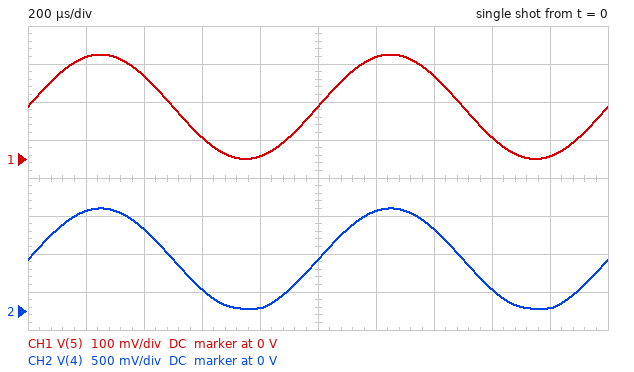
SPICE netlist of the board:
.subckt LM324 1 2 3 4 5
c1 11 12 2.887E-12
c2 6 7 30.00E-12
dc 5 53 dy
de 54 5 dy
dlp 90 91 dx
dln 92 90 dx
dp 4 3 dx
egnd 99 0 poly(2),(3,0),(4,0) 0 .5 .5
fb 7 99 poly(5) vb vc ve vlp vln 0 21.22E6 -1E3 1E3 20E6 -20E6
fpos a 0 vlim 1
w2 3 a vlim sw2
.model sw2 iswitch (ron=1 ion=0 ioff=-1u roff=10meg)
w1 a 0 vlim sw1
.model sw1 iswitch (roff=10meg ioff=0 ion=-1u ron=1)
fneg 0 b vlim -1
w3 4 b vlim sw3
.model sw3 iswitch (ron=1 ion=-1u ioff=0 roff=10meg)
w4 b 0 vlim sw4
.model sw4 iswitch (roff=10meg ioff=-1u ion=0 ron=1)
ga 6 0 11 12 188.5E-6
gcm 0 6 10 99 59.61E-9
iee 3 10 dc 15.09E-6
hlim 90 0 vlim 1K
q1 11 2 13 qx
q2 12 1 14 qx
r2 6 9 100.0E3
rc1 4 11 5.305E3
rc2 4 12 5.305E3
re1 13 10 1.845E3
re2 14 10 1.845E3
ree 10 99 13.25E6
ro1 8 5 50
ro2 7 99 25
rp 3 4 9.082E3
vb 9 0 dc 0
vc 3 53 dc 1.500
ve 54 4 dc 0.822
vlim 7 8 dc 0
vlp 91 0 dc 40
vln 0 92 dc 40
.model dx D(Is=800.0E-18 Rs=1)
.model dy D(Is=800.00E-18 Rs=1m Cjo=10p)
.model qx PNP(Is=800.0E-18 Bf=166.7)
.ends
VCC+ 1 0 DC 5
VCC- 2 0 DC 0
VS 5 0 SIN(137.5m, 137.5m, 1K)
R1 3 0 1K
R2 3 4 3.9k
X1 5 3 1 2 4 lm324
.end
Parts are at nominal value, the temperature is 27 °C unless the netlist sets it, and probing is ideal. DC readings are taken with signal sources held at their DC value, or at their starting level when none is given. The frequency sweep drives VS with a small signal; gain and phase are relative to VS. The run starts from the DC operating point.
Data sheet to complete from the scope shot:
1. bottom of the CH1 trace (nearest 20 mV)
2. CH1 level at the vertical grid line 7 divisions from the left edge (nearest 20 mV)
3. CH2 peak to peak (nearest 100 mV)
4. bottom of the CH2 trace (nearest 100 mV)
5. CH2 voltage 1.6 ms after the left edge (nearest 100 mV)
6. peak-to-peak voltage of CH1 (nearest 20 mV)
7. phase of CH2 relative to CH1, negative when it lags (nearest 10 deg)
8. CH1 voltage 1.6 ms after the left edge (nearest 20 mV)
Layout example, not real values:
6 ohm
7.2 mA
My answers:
0 V
220 mV
1.3 V
0 V
300 mV
280 mV
0 deg
60 mV
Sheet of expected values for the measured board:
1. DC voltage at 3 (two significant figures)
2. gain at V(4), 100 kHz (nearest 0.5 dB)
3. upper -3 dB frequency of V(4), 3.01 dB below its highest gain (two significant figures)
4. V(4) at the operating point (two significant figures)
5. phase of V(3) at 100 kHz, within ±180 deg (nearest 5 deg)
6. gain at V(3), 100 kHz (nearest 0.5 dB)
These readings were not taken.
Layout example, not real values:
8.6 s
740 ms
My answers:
140 mV
13.0 dB
210 kHz
680 mV
-25 deg
-1.0 dB
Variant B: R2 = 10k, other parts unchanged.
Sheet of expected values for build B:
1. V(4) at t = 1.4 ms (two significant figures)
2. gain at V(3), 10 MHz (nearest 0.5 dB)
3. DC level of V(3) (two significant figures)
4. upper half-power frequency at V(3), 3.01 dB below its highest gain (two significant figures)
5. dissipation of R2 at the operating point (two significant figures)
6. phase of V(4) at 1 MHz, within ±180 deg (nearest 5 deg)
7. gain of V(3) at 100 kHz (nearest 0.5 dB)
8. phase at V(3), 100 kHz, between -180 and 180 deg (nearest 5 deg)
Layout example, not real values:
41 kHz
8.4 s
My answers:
2.4 V
-48.5 dB
140 mV
93 kHz
190 µW
-95 deg
-3.5 dB
-50 deg
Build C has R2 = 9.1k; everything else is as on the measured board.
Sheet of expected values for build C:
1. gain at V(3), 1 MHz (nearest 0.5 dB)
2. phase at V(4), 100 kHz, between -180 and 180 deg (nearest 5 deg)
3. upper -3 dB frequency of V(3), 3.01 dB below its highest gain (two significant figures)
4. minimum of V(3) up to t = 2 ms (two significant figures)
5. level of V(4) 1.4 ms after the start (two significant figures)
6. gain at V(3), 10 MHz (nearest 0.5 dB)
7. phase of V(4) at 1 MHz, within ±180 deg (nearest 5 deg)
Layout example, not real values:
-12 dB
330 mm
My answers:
-20.0 dB
-45 deg
100 kHz
4.0 mV
2.2 V
-47.5 dB
-95 deg
